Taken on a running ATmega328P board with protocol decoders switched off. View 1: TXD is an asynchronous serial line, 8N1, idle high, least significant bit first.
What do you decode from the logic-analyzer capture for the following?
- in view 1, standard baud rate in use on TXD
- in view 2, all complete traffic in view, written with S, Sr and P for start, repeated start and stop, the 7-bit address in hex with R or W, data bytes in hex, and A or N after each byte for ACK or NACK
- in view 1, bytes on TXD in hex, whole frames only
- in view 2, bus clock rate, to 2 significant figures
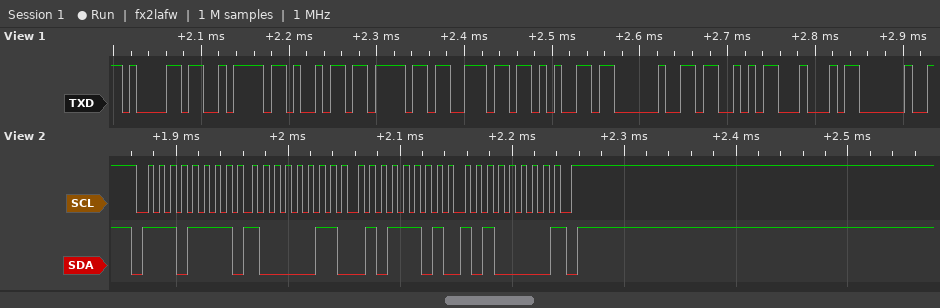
115200 baud
S 77R A 83 A 5D A A0 N P
0x61 0x7A 0x69 0x6F 0x6E 0x65 0x20 0x53 0x44 0x20
100 kHz
